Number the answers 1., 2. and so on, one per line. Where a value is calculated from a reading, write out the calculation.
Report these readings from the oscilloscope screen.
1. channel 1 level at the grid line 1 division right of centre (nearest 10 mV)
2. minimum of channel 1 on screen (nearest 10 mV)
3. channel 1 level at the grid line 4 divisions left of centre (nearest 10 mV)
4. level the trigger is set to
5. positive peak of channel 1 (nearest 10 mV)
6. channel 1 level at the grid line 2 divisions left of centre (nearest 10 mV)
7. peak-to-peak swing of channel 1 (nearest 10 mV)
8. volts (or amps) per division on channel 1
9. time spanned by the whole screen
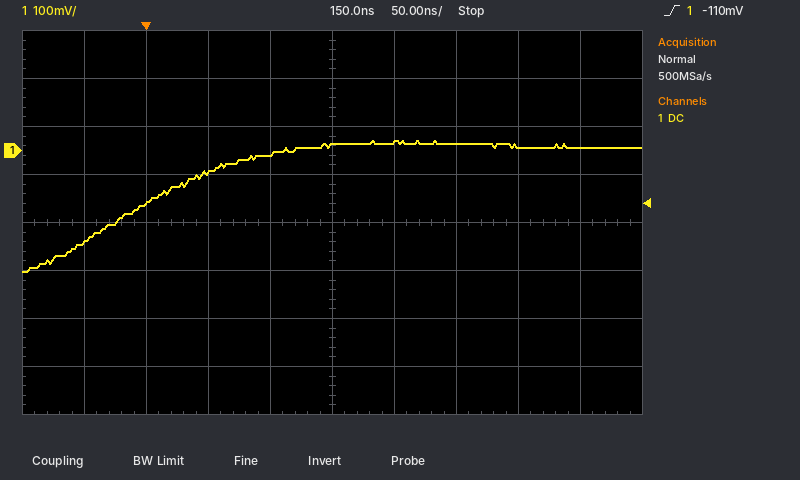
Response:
1. 20 mV
2. -250 mV
3. -190 mV
4. -110 mV
5. 20 mV
6. -50 mV
7. 20 mV − (-250 mV) = 270 mV
8. 100 mV
9. 500 ns
